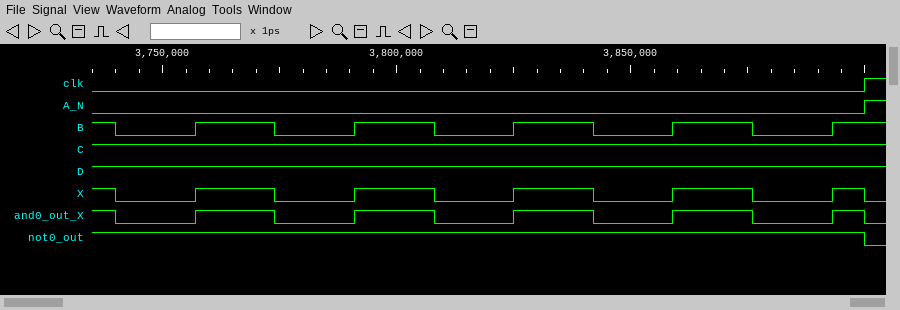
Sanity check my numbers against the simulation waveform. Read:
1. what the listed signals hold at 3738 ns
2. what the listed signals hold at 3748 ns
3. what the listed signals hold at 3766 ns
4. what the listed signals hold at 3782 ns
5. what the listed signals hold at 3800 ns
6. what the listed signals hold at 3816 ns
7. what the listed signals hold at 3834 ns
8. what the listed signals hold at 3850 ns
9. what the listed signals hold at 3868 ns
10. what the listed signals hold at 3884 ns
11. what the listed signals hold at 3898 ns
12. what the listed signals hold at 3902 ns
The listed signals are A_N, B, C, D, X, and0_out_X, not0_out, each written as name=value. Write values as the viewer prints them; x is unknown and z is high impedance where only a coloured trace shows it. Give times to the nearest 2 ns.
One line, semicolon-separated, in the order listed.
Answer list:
A_N=0, B=1, C=1, D=1, X=1, and0_out_X=1, not0_out=1; A_N=0, B=0, C=1, D=1, X=0, and0_out_X=0, not0_out=1; A_N=0, B=1, C=1, D=1, X=1, and0_out_X=1, not0_out=1; A_N=0, B=0, C=1, D=1, X=0, and0_out_X=0, not0_out=1; A_N=0, B=1, C=1, D=1, X=1, and0_out_X=1, not0_out=1; A_N=0, B=0, C=1, D=1, X=0, and0_out_X=0, not0_out=1; A_N=0, B=1, C=1, D=1, X=1, and0_out_X=1, not0_out=1; A_N=0, B=0, C=1, D=1, X=0, and0_out_X=0, not0_out=1; A_N=0, B=1, C=1, D=1, X=1, and0_out_X=1, not0_out=1; A_N=0, B=0, C=1, D=1, X=0, and0_out_X=0, not0_out=1; A_N=0, B=1, C=1, D=1, X=1, and0_out_X=1, not0_out=1; A_N=1, B=1, C=1, D=1, X=0, and0_out_X=0, not0_out=0
